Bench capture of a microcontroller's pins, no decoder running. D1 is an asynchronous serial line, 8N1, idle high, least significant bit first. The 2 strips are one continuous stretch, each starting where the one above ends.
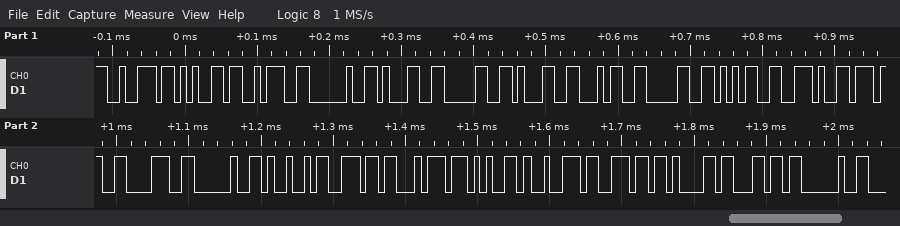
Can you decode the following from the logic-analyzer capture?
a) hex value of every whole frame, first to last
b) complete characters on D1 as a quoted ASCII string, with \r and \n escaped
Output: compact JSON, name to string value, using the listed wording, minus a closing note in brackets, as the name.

{"hex value of every whole frame, first to last": "72 65 3A 20 31 30 31 34 30 35 2E 37 38 20 49 6E 74 65 72 6E 61 6C 20", "complete characters on D1 as a quoted ASCII string, with \\r and \\n escaped": "\"re: 101405.78 Internal \""}
